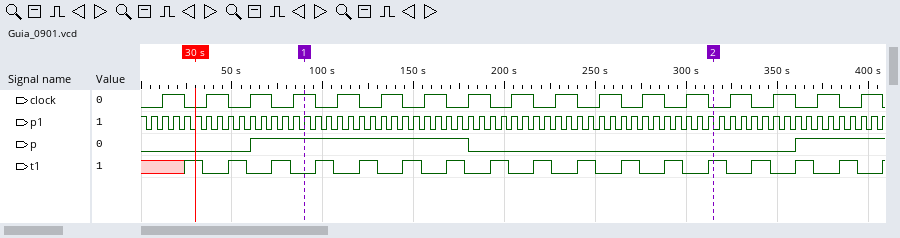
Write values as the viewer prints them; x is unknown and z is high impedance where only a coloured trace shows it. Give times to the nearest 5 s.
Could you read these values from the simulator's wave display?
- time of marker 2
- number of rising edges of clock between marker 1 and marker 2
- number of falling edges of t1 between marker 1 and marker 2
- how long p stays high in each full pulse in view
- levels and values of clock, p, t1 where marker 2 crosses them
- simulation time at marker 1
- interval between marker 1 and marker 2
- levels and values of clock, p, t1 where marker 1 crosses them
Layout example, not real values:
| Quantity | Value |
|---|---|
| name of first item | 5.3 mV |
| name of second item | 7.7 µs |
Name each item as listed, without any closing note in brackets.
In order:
| Quantity | Value |
|---|---|
| time of marker 2 | 315 s |
| number of rising edges of clock between marker 1 and marker 2 | 9 |
| number of falling edges of t1 between marker 1 and marker 2 | 9 |
| how long p stays high in each full pulse in view | 120 s |
| levels and values of clock, p, t1 where marker 2 crosses them | clock=0, p=0, t1=1 |
| simulation time at marker 1 | 90 s |
| interval between marker 1 and marker 2 | 225 s |
| levels and values of clock, p, t1 where marker 1 crosses them | clock=1, p=1, t1=0 |
